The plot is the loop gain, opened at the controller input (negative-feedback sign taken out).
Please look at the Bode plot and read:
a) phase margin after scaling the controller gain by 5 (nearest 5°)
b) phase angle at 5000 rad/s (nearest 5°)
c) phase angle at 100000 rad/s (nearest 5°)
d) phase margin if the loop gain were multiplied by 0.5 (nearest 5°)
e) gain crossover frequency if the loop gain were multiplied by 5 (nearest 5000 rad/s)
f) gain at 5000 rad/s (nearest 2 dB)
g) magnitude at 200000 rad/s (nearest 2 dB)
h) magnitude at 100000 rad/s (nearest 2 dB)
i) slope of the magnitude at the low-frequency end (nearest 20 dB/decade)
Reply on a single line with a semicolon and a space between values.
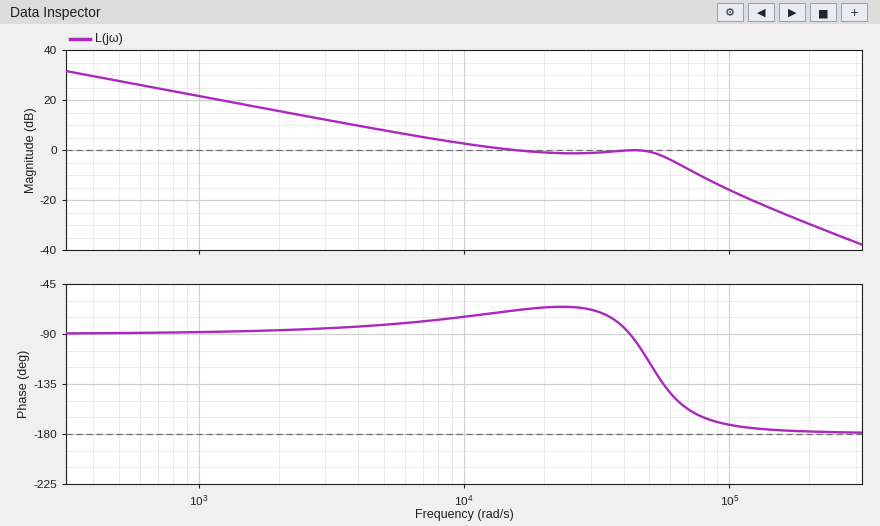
10°; -80°; -170°; 100°; 90000 rad/s; 8 dB; -30 dB; -16 dB; -20 dB/decade
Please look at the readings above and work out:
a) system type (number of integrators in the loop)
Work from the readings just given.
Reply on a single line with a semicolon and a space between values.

1
